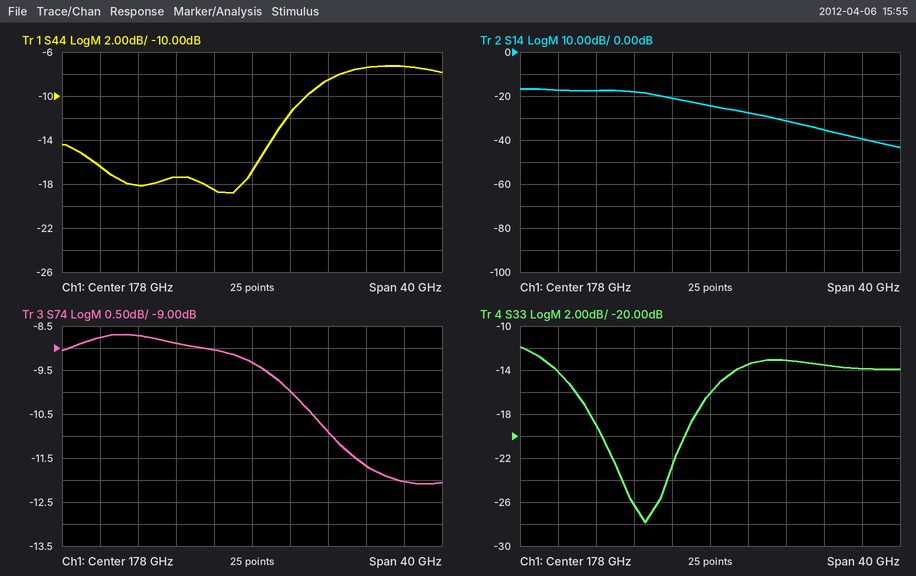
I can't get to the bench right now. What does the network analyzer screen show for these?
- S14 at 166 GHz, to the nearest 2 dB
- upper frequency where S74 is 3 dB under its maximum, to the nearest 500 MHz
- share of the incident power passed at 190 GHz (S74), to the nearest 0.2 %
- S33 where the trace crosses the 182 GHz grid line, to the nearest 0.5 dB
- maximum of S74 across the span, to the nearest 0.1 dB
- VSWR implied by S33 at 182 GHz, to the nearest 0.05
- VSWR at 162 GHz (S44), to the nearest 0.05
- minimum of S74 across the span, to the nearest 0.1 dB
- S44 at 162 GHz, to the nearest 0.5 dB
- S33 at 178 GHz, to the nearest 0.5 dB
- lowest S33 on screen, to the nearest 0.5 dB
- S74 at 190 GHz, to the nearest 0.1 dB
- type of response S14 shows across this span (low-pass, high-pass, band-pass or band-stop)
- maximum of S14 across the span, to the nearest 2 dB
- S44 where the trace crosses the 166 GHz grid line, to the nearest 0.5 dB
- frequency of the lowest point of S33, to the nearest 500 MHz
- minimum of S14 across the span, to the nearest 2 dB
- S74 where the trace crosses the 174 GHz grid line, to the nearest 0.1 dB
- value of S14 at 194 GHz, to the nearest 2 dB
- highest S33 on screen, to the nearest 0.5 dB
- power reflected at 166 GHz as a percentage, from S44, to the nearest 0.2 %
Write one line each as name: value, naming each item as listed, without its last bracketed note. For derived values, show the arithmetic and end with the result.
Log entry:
S14 at 166 GHz, to the nearest 2 dB: -18 dB
upper frequency where S74 is 3 dB under its maximum, to the nearest 500 MHz: 190.0 GHz
share of the incident power passed at 190 GHz (S74), to the nearest 0.2 %: 10^(-11.7/10) ≈ 6.8 %
S33 where the trace crosses the 182 GHz grid line, to the nearest 0.5 dB: -13.5 dB
maximum of S74 across the span, to the nearest 0.1 dB: -8.7 dB
VSWR implied by S33 at 182 GHz, to the nearest 0.05: |Γ| = 10^(-13.5/20) = 0.2113; VSWR = (1 + 0.2113)/(1 − 0.2113) ≈ 1.54, so 1.55 to the nearest 0.05
VSWR at 162 GHz (S44), to the nearest 0.05: |Γ| = 10^(-16.5/20) = 0.1496; VSWR = (1 + 0.1496)/(1 − 0.1496) ≈ 1.35
minimum of S74 across the span, to the nearest 0.1 dB: -12.1 dB
S44 at 162 GHz, to the nearest 0.5 dB: -16.5 dB
S33 at 178 GHz, to the nearest 0.5 dB: -16.0 dB
lowest S33 on screen, to the nearest 0.5 dB: -28.0 dB
S74 at 190 GHz, to the nearest 0.1 dB: -11.7 dB
type of response S14 shows across this span: low-pass
maximum of S14 across the span, to the nearest 2 dB: -16 dB
S44 where the trace crosses the 166 GHz grid line, to the nearest 0.5 dB: -18.0 dB
frequency of the lowest point of S33, to the nearest 500 MHz: 171.0 GHz
minimum of S14 across the span, to the nearest 2 dB: -44 dB
S74 where the trace crosses the 174 GHz grid line, to the nearest 0.1 dB: -9.0 dB
value of S14 at 194 GHz, to the nearest 2 dB: -40 dB
highest S33 on screen, to the nearest 0.5 dB: -12.0 dB
power reflected at 166 GHz as a percentage, from S44, to the nearest 0.2 %: 10^(-18/10) ≈ 1.6 %
